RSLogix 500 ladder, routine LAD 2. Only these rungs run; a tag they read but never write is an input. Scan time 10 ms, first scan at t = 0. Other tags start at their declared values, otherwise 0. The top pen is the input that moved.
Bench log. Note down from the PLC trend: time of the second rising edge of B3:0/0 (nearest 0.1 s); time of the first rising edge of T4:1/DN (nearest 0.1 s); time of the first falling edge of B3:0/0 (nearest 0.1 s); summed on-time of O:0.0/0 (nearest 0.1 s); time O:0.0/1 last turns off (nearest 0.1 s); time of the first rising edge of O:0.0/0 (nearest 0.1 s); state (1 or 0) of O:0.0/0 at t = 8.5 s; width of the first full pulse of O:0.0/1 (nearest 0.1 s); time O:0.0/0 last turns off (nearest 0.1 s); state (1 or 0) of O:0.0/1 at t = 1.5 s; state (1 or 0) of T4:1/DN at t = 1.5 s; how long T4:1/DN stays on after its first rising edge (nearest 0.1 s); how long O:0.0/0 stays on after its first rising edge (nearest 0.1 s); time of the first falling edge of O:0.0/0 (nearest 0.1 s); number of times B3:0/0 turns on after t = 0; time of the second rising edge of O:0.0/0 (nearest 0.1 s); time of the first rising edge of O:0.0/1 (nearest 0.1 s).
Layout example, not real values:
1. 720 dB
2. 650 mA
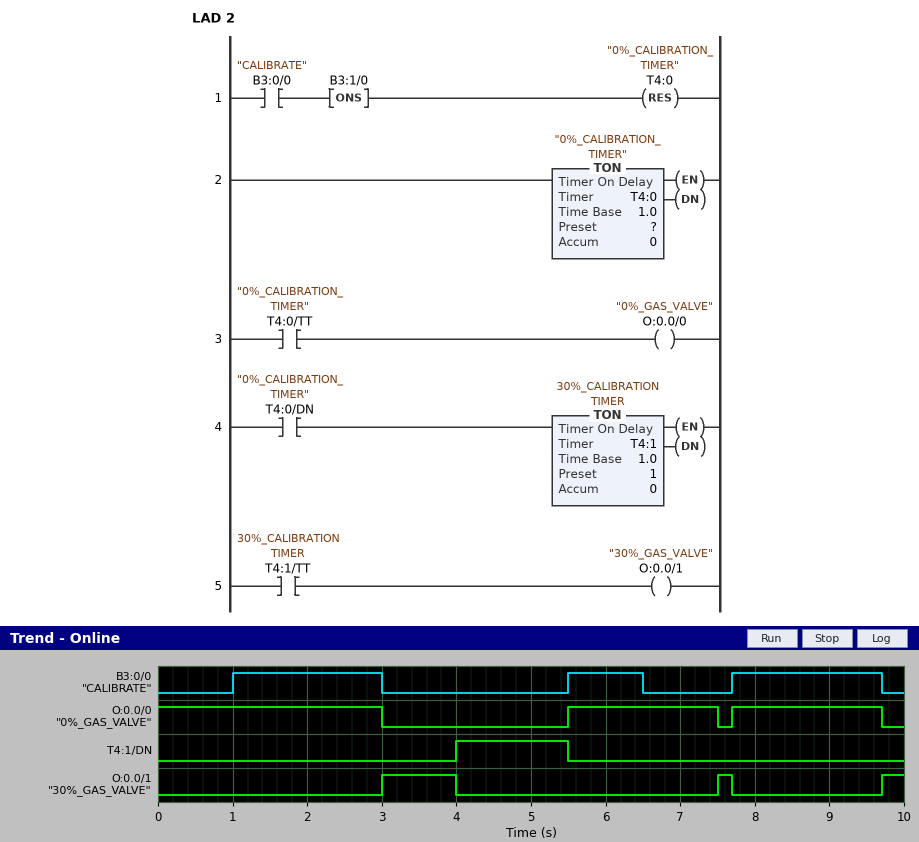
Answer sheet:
1. 5.5 s
2. 4.0 s
3. 3.0 s
4. 7.0 s
5. 7.7 s
6. 5.5 s
7. 1
8. 1.0 s
9. 9.7 s
10. 0
11. 0
12. 1.5 s
13. 2.0 s
14. 3.0 s
15. 3
16. 7.7 s
17. 3.0 s
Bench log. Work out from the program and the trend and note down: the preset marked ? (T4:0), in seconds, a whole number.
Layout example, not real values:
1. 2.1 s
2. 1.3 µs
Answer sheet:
1. 2 s
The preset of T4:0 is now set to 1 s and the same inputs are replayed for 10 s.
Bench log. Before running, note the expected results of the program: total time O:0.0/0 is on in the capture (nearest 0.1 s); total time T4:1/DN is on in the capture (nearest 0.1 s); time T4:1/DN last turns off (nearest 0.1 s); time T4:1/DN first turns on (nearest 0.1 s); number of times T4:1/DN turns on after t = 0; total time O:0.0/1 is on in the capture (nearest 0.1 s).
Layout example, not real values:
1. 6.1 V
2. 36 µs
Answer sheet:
1. 4.0 s
2. 3.0 s
3. 7.7 s
4. 3.0 s
5. 3
6. 3.0 s
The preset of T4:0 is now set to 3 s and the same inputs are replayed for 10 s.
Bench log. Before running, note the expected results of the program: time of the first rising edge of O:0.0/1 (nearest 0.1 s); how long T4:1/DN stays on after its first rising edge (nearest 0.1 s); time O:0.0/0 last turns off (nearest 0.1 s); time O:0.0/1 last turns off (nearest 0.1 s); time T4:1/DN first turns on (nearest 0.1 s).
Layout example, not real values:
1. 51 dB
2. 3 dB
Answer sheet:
1. 4.0 s
2. 0.5 s
3. 4.0 s
4. 5.0 s
5. 5.0 s
